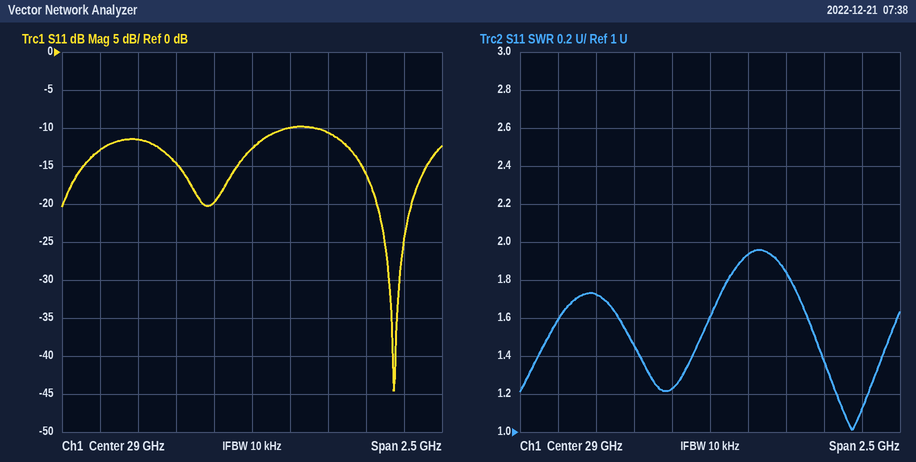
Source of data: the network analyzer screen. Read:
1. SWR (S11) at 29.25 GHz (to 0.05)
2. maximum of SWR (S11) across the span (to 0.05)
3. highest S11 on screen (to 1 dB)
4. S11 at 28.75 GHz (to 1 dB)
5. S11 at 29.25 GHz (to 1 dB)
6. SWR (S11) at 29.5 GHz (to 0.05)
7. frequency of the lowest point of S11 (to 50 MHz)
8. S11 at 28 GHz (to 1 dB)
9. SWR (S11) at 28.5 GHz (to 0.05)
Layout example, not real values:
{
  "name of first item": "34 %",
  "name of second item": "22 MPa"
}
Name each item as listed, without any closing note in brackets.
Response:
{
  "SWR (S11) at 29.25 GHz": "1.95",
  "maximum of SWR (S11) across the span": "1.95",
  "highest S11 on screen": "-10 dB",
  "S11 at 28.75 GHz": "-20 dB",
  "S11 at 29.25 GHz": "-10 dB",
  "SWR (S11) at 29.5 GHz": "1.85",
  "frequency of the lowest point of S11": "29.95 GHz",
  "S11 at 28 GHz": "-13 dB",
  "SWR (S11) at 28.5 GHz": "1.45"
}
